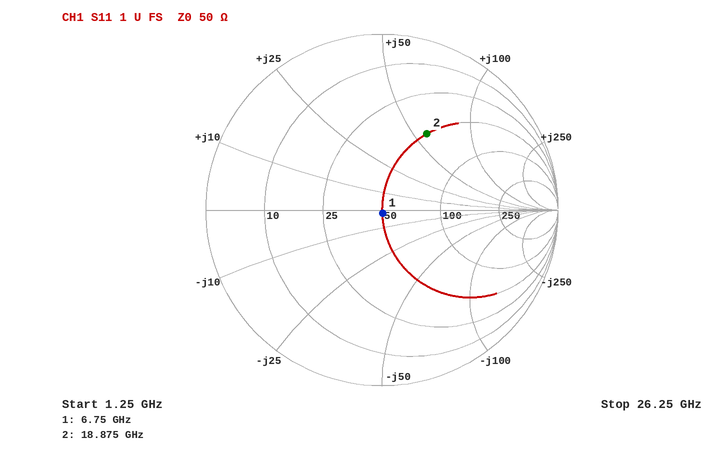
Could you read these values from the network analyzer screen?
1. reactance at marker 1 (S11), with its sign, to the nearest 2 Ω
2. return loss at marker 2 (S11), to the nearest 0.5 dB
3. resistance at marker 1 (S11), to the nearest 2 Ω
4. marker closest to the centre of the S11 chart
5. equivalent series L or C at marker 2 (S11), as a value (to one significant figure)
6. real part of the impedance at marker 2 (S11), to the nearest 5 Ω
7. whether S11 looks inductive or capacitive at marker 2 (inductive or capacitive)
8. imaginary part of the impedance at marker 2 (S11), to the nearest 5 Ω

-2 Ω
6.0 dB
50 Ω
marker 1
500 pH
50 Ω
inductive
+60 Ω
